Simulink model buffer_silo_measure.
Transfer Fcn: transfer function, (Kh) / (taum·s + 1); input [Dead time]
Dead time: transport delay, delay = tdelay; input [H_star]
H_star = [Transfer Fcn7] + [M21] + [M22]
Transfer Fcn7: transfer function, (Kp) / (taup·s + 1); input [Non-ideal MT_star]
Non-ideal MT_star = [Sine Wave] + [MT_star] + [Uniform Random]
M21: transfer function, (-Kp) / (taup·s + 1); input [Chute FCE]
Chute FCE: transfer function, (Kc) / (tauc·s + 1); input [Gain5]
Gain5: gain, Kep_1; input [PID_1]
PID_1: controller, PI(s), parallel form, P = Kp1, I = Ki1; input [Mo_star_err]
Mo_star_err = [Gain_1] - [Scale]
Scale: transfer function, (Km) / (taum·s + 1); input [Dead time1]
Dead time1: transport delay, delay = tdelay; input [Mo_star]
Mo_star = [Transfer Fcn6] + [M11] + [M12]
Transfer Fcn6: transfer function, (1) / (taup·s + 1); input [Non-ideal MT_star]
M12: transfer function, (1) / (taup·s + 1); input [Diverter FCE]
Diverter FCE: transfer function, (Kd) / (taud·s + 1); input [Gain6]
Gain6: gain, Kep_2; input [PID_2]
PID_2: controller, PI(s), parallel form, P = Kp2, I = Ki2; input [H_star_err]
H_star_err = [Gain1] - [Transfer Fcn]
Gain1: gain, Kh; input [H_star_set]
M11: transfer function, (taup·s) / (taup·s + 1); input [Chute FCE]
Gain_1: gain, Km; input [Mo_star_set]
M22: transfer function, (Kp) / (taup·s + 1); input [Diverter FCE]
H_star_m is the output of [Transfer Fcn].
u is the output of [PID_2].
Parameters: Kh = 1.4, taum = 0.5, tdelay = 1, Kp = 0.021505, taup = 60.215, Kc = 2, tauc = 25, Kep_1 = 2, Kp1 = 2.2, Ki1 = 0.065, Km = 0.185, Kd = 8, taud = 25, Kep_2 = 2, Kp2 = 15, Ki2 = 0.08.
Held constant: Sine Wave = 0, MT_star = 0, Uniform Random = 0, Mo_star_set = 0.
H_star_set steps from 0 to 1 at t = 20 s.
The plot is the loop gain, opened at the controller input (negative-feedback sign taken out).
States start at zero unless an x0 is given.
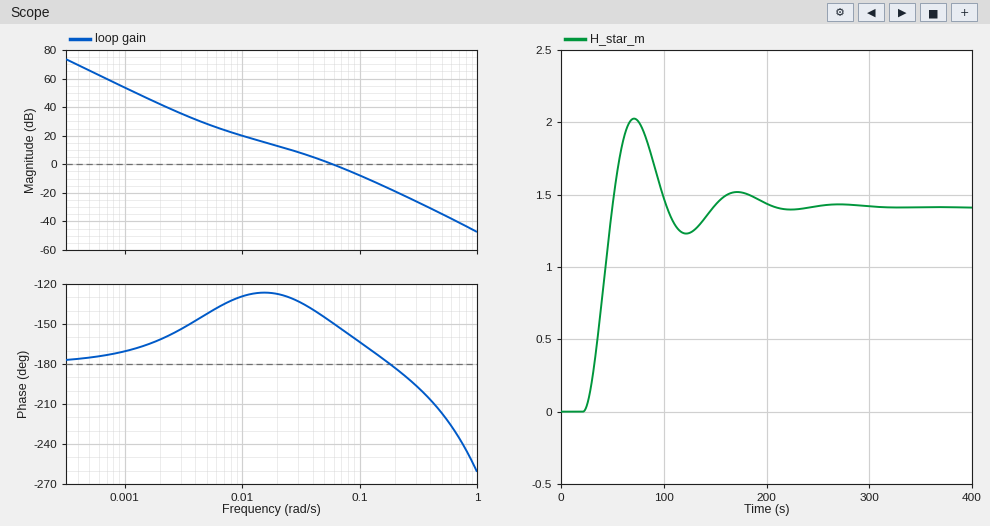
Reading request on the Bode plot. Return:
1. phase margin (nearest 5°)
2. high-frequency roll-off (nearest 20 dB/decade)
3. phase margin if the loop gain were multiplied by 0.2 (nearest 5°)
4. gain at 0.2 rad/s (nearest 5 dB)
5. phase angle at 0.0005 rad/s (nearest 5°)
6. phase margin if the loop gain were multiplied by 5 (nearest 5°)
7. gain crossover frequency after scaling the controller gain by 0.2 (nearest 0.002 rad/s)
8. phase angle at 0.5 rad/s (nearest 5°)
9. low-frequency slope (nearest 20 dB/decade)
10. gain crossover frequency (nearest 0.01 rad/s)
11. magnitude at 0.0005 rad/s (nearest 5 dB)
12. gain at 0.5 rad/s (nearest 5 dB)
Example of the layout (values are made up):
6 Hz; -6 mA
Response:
30°; -40 dB/decade; 55°; -20 dB; -175°; 5°; 0.018 rad/s; -215°; -40 dB/decade; 0.06 rad/s; 65 dB; -35 dB
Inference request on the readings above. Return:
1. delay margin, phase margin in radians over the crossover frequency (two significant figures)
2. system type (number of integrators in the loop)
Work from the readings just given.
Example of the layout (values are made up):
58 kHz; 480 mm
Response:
8.7 s; 2
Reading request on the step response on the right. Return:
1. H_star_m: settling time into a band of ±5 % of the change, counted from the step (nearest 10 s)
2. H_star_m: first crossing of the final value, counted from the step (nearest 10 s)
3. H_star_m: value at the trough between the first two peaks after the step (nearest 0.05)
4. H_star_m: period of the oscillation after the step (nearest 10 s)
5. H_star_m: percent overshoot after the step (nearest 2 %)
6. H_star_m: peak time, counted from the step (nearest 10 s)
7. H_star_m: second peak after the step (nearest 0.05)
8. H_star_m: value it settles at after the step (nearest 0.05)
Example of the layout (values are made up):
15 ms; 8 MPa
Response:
170 s; 30 s; 1.25; 100 s; 44 %; 50 s; 1.50; 1.40
